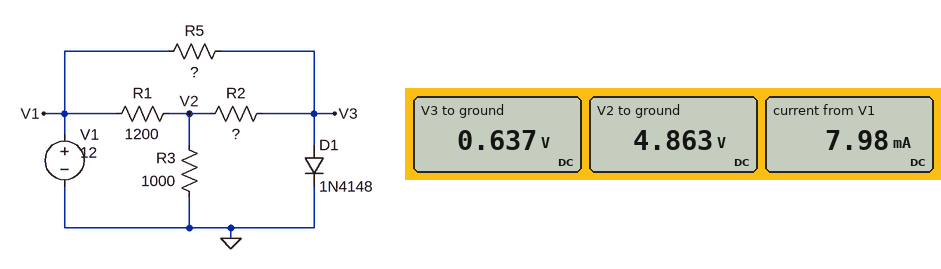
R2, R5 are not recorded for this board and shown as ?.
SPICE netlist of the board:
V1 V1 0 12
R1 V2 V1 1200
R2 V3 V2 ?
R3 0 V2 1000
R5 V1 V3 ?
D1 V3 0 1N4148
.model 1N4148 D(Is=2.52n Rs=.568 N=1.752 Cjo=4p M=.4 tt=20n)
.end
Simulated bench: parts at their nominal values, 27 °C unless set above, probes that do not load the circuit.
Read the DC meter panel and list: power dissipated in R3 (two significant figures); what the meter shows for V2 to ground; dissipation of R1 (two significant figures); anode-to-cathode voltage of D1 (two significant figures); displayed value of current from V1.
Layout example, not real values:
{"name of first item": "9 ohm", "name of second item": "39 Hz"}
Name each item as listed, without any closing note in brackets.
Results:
{"power dissipated in R3": "24 mW", "what the meter shows for V2 to ground": "4.863 V", "dissipation of R1": "42 mW", "anode-to-cathode voltage of D1": "640 mV", "displayed value of current from V1": "7.98 mA"}
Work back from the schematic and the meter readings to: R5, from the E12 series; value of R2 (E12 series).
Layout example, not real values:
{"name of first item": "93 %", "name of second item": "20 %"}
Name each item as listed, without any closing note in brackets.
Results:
{"R5, from the E12 series": "5.6 kΩ", "value of R2": "3.9 kΩ"}
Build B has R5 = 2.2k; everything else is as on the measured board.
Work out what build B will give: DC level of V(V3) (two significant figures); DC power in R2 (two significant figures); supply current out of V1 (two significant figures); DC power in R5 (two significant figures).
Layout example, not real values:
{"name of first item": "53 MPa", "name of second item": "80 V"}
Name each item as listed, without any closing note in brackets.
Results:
{"DC level of V(V3)": "670 mV", "DC power in R2": "4.5 mW", "supply current out of V1": "11 mA", "DC power in R5": "58 mW"}
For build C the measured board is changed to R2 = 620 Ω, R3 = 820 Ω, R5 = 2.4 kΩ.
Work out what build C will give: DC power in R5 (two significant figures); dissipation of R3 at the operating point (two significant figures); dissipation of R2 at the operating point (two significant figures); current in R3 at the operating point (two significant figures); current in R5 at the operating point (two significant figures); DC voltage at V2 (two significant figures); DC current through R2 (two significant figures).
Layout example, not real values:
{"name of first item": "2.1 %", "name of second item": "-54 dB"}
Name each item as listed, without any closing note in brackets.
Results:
{"DC power in R5": "53 mW", "dissipation of R3 at the operating point": "11 mW", "dissipation of R2 at the operating point": "8.9 mW", "current in R3 at the operating point": "3.7 mA", "current in R5 at the operating point": "4.7 mA", "DC voltage at V2": "3.0 V", "DC current through R2": "3.8 mA"}
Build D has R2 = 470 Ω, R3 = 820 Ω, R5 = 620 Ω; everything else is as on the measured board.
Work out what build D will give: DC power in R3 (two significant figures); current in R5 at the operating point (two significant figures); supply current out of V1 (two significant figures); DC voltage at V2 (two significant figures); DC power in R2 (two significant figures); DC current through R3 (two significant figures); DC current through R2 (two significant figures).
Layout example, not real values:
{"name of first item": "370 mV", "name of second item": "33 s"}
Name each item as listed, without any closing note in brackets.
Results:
{"DC power in R3": "9.3 mW", "current in R5 at the operating point": "18 mA", "supply current out of V1": "26 mA", "DC voltage at V2": "2.8 V", "DC power in R2": "8.8 mW", "DC current through R3": "3.4 mA", "DC current through R2": "4.3 mA"}
